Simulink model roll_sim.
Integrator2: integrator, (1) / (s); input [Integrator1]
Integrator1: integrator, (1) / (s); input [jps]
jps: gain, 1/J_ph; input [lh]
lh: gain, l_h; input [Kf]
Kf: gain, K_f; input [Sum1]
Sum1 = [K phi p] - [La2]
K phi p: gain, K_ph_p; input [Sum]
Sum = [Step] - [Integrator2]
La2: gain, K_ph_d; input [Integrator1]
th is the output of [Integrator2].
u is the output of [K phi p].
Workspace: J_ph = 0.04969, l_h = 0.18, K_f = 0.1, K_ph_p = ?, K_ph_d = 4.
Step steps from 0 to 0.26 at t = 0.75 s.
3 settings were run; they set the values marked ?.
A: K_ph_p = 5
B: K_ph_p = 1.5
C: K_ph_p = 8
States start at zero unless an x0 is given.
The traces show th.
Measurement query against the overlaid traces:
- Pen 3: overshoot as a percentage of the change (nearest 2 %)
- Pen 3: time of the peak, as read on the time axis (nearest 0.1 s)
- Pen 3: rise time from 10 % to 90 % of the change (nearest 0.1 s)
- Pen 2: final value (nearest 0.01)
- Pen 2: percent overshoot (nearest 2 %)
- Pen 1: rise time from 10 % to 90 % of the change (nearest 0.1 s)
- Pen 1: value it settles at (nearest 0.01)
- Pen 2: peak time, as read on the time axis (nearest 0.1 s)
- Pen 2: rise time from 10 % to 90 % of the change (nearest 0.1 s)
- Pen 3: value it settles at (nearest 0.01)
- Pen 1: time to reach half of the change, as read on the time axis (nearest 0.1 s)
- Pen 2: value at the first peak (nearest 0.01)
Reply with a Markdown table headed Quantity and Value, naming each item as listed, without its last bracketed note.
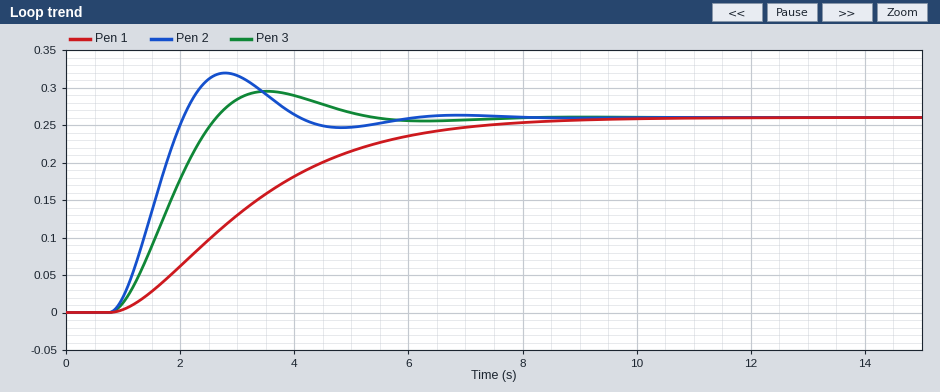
| Quantity | Value |
|---|---|
| Pen 3: overshoot as a percentage of the change | 14 % |
| Pen 3: time of the peak, as read on the time axis | 3.5 s |
| Pen 3: rise time from 10 % to 90 % of the change | 1.3 s |
| Pen 2: final value | 0.26 |
| Pen 2: percent overshoot | 22 % |
| Pen 1: rise time from 10 % to 90 % of the change | 4.4 s |
| Pen 1: value it settles at | 0.26 |
| Pen 2: peak time, as read on the time axis | 2.8 s |
| Pen 2: rise time from 10 % to 90 % of the change | 0.9 s |
| Pen 3: value it settles at | 0.26 |
| Pen 1: time to reach half of the change, as read on the time axis | 3.0 s |
| Pen 2: value at the first peak | 0.32 |
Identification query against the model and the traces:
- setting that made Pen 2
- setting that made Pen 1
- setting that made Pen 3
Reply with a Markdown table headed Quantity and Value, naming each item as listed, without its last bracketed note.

| Quantity | Value |
|---|---|
| setting that made Pen 2 | C |
| setting that made Pen 1 | B |
| setting that made Pen 3 | A |
